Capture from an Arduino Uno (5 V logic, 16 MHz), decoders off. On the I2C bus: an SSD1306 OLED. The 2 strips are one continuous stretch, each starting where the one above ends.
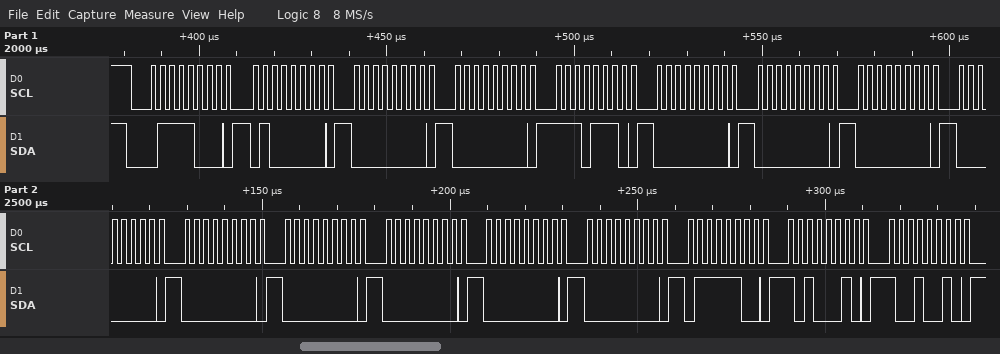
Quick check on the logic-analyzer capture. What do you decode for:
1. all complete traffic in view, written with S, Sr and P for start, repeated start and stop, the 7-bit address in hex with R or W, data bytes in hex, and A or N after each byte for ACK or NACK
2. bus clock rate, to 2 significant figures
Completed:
S 3CW A 40 A 00 A 00 A EE A 00 A 00 A 00 A 00 A 00 A 00 A 00 A 00 A 00 A 7C A A2 A 92 A
400 kHz
